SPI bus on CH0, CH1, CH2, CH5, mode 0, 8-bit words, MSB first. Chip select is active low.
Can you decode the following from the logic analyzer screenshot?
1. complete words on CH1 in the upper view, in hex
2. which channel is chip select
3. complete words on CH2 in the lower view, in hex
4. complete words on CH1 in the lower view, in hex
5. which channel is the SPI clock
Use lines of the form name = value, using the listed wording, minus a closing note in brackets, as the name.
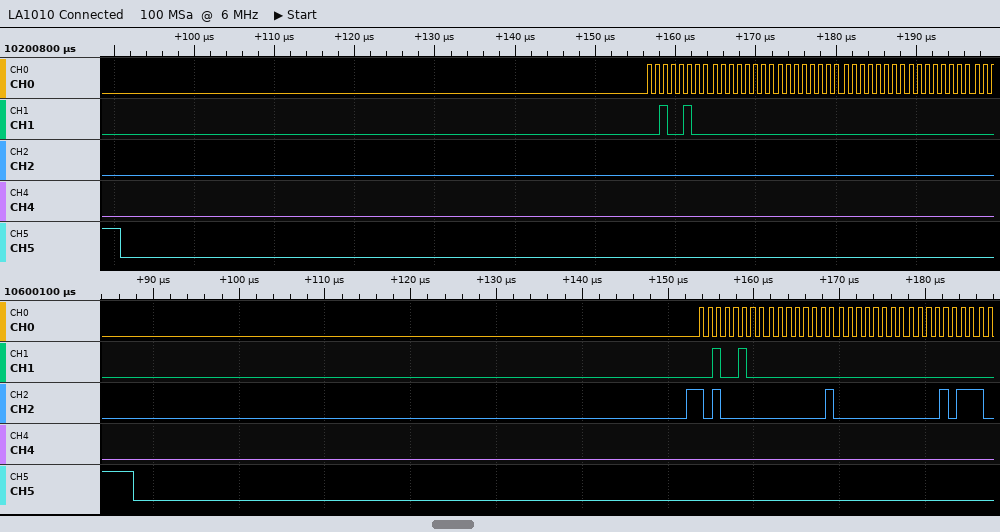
complete words on CH1 in the upper view, in hex = 24, 00, 00, 00, 00
which channel is chip select = CH5
complete words on CH2 in the lower view, in hex = A0, 01, 00, 0B
complete words on CH1 in the lower view, in hex = 24, 00, 00, 00
which channel is the SPI clock = CH0
